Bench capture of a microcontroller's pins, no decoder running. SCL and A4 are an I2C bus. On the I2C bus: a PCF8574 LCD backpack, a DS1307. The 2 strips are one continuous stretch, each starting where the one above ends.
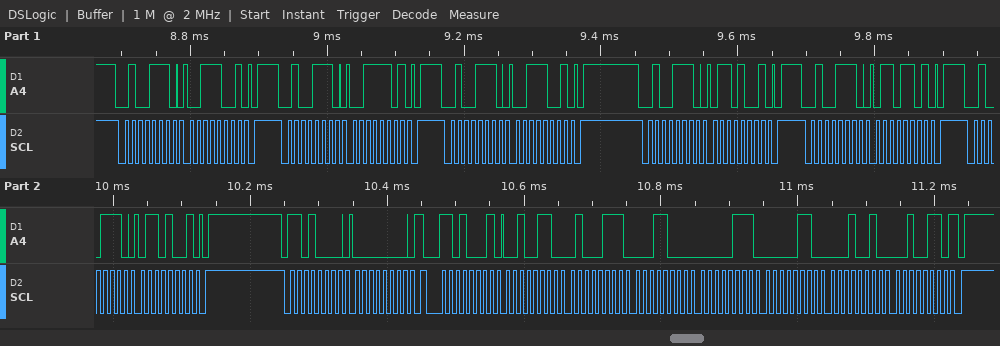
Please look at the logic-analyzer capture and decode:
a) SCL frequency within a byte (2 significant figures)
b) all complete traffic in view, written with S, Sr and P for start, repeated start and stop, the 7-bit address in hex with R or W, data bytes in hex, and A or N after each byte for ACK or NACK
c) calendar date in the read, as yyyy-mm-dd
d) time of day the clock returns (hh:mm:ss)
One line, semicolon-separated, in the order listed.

100 kHz; S 27W A 39 A P S 27W A 3D A P S 27W A 39 A P S 27W A 69 A P S 27W A 6D A P S 27W A 69 A P S 68W A 00 A Sr 68R A 26 A 47 A 18 A 07 A 06 A 12 A 26 N P; 2026-12-06; 18:47:26
